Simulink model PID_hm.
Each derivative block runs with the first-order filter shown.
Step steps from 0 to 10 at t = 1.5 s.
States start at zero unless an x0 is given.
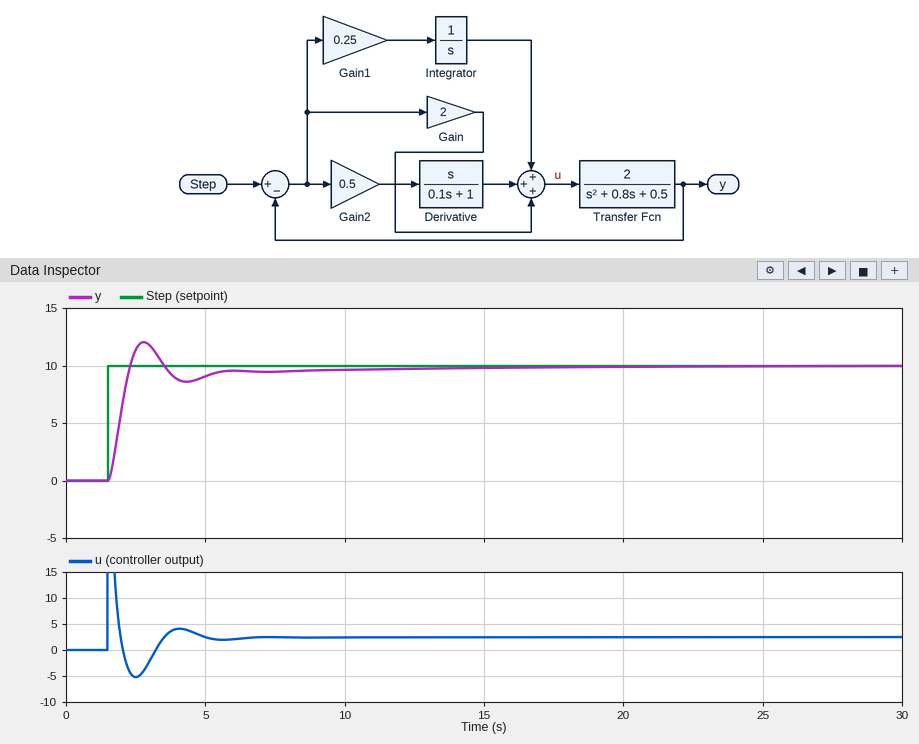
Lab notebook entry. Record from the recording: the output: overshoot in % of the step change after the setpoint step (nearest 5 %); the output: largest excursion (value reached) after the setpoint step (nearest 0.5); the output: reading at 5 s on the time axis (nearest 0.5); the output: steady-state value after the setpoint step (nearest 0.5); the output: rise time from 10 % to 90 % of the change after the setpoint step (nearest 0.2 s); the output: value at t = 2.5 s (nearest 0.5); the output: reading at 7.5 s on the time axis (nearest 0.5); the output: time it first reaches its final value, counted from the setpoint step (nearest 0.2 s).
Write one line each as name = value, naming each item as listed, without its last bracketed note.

the output: overshoot in % of the step change after the setpoint step = 20 %
the output: largest excursion (value reached) after the setpoint step = 12.0
the output: reading at 5 s on the time axis = 9.0
the output: steady-state value after the setpoint step = 10.0
the output: rise time from 10 % to 90 % of the change after the setpoint step = 0.6 s
the output: value at t = 2.5 s = 11.5
the output: reading at 7.5 s on the time axis = 9.5
the output: time it first reaches its final value, counted from the setpoint step = 0.8 s
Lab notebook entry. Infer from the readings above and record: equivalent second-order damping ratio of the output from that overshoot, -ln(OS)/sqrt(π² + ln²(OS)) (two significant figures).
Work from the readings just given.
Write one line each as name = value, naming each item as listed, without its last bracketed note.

equivalent second-order damping ratio of the output from that overshoot, -ln(OS)/sqrt(π² + ln²(OS)) = 0.46
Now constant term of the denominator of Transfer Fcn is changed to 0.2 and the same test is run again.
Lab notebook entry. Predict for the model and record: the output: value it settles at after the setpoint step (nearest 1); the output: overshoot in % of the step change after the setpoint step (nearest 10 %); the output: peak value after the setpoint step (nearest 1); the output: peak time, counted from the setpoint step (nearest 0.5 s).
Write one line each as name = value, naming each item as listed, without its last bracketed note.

the output: value it settles at after the setpoint step = 10
the output: overshoot in % of the step change after the setpoint step = 30 %
the output: peak value after the setpoint step = 13
the output: peak time, counted from the setpoint step = 1.5 s
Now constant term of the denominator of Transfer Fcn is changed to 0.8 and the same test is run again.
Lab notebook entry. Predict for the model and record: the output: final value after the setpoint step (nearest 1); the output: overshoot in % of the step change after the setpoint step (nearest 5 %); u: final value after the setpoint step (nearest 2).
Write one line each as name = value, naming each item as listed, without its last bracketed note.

the output: final value after the setpoint step = 10
the output: overshoot in % of the step change after the setpoint step = 15 %
u: final value after the setpoint step = 4
